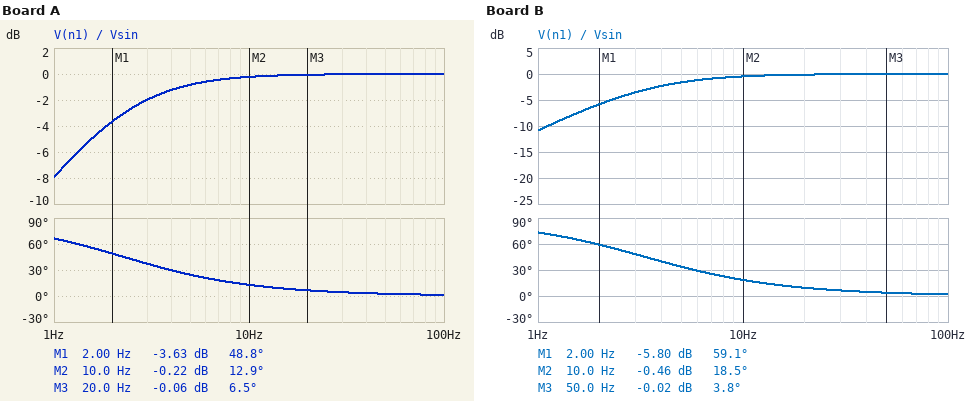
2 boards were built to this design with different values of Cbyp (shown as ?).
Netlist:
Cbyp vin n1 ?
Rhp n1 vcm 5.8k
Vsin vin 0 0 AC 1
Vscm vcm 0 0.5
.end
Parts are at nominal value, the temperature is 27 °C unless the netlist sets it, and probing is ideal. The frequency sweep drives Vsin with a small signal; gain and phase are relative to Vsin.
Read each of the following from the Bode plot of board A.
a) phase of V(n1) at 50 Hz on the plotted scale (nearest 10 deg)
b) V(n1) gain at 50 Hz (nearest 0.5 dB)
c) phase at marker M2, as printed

0 deg
0 dB
12.9 deg
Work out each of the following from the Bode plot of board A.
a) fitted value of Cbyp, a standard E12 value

12 µF
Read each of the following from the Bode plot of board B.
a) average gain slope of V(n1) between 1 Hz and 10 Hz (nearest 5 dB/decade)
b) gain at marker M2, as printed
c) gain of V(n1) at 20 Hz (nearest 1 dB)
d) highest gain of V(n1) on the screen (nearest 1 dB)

10 dB/decade
-0.46 dB
0 dB
0 dB
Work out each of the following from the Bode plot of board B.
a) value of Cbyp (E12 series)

8.2 µF
